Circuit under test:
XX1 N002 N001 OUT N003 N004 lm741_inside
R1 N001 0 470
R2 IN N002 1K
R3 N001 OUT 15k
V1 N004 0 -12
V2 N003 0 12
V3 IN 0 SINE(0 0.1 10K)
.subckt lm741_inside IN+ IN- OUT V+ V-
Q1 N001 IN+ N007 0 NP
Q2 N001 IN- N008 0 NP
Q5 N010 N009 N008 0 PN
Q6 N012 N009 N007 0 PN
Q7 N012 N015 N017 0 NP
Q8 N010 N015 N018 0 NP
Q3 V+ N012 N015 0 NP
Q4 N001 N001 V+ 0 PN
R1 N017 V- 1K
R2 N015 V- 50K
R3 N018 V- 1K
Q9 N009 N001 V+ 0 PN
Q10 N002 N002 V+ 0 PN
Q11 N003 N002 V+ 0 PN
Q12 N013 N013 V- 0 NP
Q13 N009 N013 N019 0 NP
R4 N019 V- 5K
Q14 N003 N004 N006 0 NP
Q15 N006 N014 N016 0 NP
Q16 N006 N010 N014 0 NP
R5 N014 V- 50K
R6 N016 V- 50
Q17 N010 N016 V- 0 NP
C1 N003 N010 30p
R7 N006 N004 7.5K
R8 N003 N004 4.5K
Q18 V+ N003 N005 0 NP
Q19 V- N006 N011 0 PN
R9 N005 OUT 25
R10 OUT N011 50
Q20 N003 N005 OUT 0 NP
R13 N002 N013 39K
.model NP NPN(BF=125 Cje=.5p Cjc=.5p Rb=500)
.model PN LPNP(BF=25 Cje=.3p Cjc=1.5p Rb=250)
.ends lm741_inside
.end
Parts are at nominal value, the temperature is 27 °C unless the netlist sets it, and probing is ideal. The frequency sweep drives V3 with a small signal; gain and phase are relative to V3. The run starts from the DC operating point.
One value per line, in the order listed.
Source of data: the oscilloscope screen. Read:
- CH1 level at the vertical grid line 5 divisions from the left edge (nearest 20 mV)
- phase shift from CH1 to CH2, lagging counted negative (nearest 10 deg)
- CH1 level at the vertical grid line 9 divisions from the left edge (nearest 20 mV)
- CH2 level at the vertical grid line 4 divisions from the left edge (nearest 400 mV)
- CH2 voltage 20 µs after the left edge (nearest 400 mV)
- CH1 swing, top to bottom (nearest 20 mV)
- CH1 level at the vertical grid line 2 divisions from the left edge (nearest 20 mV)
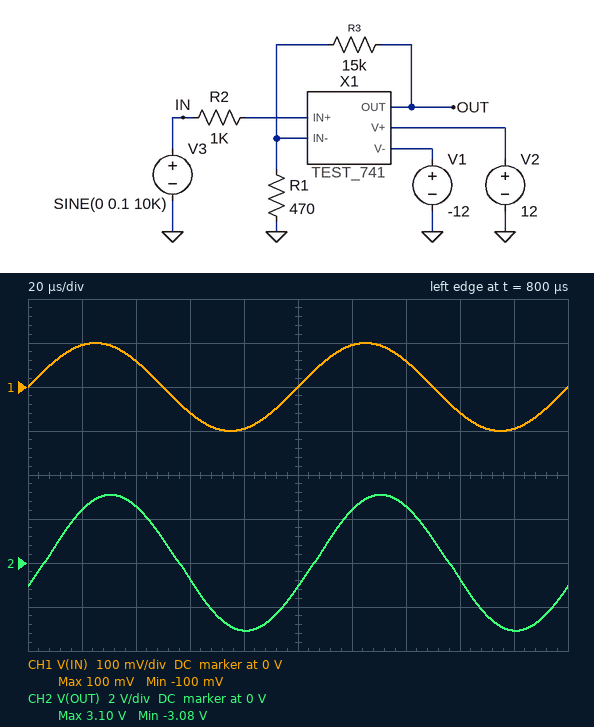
0 V
-20 deg
-100 mV
-3.2 V
2.4 V
200 mV
60 mV
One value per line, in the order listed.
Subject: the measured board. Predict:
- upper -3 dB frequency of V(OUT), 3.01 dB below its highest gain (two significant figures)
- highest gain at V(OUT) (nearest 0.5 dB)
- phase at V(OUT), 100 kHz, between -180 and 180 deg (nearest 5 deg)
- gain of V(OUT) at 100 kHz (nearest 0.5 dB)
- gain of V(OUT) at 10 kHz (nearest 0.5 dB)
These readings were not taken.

19 kHz
30.5 dB
-80 deg
16.0 dB
29.5 dB
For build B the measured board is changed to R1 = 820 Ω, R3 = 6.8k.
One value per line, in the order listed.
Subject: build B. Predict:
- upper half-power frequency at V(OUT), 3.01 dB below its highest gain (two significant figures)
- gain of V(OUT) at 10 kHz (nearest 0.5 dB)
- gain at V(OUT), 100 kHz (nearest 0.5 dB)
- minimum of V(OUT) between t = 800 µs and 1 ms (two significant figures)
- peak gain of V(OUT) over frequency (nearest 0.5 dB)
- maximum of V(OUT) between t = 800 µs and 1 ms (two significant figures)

52 kHz
19.0 dB
12.5 dB
-920 mV
19.5 dB
930 mV
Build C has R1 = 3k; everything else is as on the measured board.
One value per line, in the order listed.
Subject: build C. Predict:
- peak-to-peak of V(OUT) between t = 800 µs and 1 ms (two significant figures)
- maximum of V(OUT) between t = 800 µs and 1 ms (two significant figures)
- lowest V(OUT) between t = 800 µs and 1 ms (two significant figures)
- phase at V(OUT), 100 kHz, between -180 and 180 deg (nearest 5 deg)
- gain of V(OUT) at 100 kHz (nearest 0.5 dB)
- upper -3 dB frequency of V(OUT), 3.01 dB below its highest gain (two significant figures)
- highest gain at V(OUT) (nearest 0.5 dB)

1.2 V
600 mV
-600 mV
-40 deg
13.0 dB
110 kHz
15.5 dB
